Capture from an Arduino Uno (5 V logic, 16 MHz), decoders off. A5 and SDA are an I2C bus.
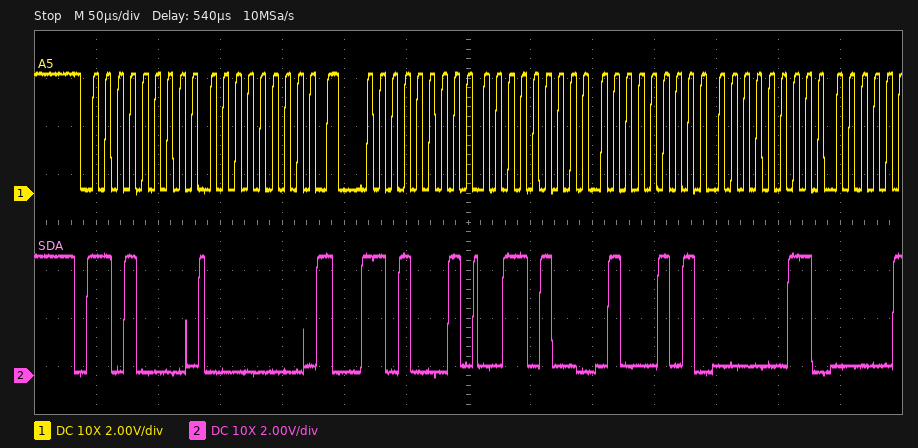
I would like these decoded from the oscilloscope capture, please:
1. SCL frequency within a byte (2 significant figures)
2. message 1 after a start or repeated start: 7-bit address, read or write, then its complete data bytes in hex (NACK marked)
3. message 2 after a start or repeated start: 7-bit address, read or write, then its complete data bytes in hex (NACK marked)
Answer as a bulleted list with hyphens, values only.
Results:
- 100 kHz
- 0x68 write: 00
- 0x68 read: 34 45 03
